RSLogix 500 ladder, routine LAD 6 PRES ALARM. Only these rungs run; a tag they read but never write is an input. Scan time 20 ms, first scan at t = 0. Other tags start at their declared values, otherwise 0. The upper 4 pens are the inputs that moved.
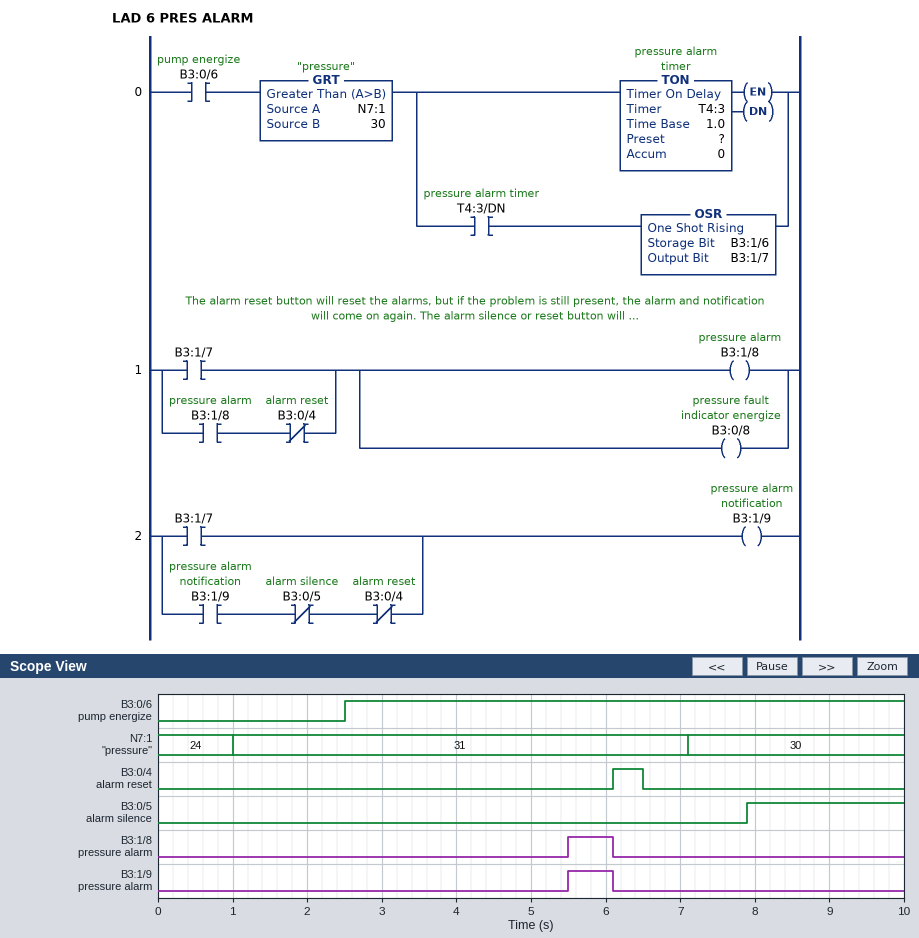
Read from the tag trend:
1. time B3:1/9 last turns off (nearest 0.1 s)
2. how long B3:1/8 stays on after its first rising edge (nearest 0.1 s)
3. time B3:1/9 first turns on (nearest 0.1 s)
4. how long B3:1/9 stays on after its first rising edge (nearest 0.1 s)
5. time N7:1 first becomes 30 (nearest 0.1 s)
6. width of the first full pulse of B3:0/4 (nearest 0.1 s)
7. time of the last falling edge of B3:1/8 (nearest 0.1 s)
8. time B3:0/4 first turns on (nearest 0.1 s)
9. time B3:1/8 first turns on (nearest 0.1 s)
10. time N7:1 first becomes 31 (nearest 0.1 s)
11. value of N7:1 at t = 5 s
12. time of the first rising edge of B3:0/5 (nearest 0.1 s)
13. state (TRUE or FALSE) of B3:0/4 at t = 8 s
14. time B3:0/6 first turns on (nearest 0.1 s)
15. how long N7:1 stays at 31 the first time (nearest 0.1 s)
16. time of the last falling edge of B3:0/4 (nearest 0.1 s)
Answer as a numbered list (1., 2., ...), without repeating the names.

1. 6.1 s
2. 0.6 s
3. 5.5 s
4. 0.6 s
5. 7.1 s
6. 0.4 s
7. 6.1 s
8. 6.1 s
9. 5.5 s
10. 1.0 s
11. 31
12. 7.9 s
13. FALSE
14. 2.5 s
15. 6.1 s
16. 6.5 s
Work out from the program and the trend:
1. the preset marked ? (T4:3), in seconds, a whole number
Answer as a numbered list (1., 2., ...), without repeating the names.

1. 3 s
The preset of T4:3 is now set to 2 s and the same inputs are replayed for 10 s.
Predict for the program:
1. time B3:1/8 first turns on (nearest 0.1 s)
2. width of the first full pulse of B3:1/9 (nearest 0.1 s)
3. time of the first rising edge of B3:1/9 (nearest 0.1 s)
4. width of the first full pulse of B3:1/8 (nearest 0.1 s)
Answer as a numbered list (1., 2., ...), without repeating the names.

1. 4.5 s
2. 1.6 s
3. 4.5 s
4. 1.6 s
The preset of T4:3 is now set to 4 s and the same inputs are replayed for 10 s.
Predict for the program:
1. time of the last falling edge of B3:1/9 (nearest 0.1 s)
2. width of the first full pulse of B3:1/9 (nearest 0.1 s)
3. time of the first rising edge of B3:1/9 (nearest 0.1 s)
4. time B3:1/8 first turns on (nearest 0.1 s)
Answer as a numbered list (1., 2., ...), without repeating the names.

1. 7.9 s
2. 1.4 s
3. 6.5 s
4. 6.5 s
